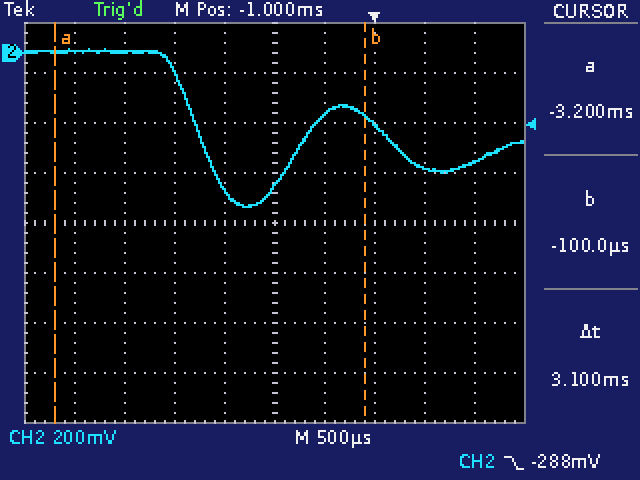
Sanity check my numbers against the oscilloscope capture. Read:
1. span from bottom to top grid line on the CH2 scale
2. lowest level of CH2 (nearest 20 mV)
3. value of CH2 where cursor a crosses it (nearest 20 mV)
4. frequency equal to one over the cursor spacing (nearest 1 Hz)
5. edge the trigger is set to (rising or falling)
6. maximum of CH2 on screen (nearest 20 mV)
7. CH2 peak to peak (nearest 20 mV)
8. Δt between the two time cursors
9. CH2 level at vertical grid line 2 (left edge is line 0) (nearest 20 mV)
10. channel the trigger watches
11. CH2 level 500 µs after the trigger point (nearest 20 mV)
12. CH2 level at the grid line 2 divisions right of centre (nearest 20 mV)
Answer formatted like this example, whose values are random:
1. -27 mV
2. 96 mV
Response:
1. 1.6 V
2. -620 mV
3. 0 mV
4. 323 Hz
5. falling
6. 20 mV
7. 640 mV
8. 3.1 ms
9. 0 mV
10. CH2
11. -460 mV
12. -280 mV
